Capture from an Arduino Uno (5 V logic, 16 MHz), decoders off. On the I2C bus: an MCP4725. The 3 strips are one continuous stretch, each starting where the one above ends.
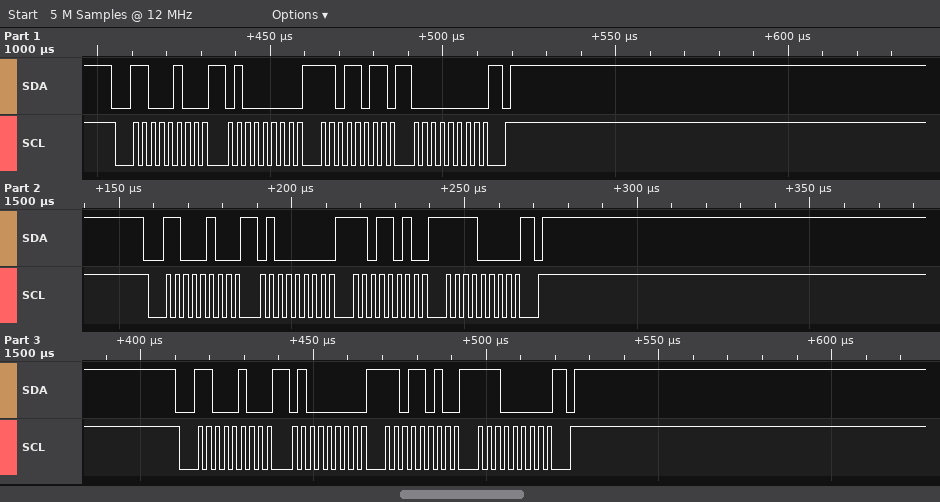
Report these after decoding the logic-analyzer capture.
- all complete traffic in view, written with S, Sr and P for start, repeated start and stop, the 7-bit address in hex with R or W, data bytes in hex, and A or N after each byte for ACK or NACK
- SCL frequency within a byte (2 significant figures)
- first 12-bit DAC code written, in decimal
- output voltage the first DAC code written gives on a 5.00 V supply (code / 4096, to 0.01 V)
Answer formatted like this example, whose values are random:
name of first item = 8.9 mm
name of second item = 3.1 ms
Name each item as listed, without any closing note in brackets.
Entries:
all complete traffic in view, written with S, Sr and P for start, repeated start and stop, the 7-bit address in hex with R or W, data bytes in hex, and A or N after each byte for ACK or NACK = S 62W A 40 A DB A 00 A P S 62W A 40 A DA A F0 A P S 62W A 40 A DA A E0 A P
SCL frequency within a byte = 400 kHz
first 12-bit DAC code written, in decimal = 3504
output voltage the first DAC code written gives on a 5.00 V supply = 4.28 V
